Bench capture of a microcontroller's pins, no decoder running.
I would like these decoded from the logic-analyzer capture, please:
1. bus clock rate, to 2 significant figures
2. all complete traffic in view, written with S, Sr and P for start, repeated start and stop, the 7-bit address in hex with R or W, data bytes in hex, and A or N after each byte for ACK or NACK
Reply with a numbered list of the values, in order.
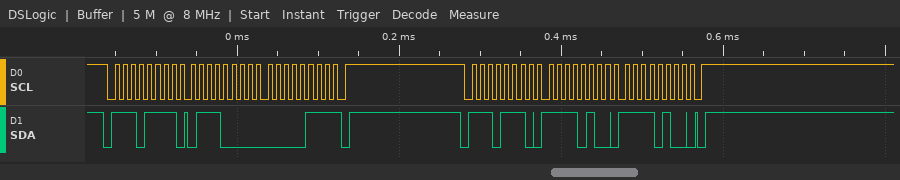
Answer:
1. 100 kHz
2. S 77R A 70 A 07 N P S 77W A F4 A F4 A P
